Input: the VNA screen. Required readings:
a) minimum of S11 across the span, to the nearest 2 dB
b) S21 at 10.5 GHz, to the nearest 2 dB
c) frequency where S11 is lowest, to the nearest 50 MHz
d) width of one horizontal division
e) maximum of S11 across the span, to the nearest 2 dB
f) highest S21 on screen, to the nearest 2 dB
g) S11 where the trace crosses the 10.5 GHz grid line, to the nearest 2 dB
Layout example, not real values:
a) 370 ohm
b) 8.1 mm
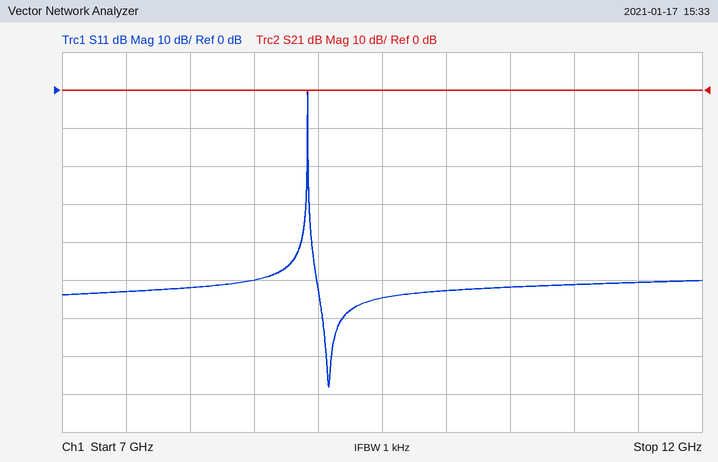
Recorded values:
a) -78 dB
b) 0 dB
c) 9.10 GHz
d) 500 MHz
e) 0 dB
f) 0 dB
g) -52 dB
